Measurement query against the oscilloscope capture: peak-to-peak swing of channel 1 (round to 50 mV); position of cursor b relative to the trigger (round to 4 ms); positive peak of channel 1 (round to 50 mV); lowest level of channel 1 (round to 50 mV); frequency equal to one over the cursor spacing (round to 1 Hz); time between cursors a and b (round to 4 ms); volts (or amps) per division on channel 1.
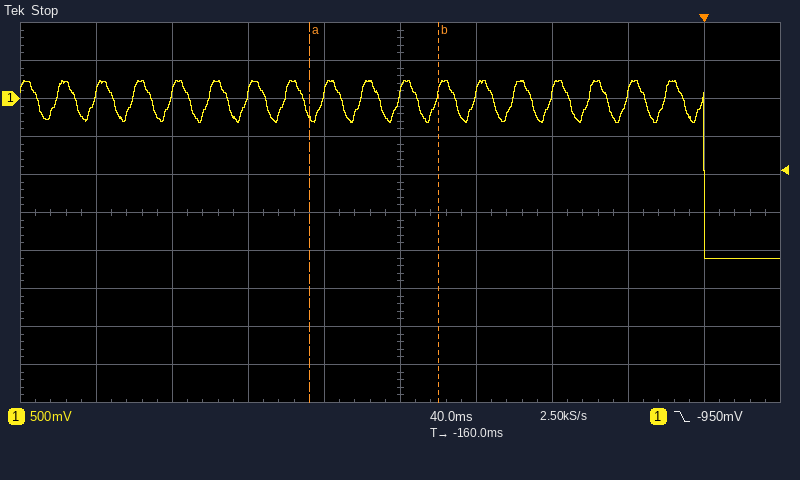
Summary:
2.35 V
-140 ms
250 mV
-2.10 V
15 Hz
68 ms
500 mV
